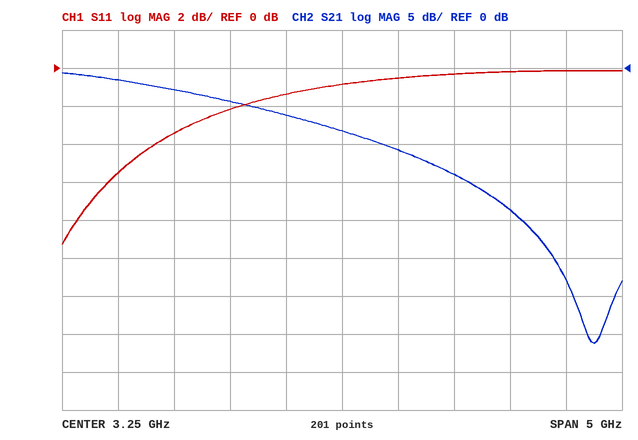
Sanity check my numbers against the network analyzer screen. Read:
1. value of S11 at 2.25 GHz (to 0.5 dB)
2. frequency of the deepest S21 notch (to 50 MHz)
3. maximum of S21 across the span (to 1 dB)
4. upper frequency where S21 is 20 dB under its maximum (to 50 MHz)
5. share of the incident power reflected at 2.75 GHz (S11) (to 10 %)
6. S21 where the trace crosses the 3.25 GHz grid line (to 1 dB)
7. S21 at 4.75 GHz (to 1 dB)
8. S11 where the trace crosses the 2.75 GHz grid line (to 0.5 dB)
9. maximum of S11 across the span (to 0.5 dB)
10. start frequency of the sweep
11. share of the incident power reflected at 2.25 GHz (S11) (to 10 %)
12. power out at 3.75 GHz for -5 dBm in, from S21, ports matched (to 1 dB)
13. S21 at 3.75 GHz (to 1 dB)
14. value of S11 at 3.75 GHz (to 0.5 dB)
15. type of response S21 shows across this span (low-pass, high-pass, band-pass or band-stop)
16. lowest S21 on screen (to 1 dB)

-2.0 dB
5.50 GHz
-1 dB
4.90 GHz
70 %
-8 dB
-19 dB
-1.5 dB
0.0 dB
750 MHz
60 %
-16 dBm
-11 dB
-0.5 dB
low-pass
-36 dB
